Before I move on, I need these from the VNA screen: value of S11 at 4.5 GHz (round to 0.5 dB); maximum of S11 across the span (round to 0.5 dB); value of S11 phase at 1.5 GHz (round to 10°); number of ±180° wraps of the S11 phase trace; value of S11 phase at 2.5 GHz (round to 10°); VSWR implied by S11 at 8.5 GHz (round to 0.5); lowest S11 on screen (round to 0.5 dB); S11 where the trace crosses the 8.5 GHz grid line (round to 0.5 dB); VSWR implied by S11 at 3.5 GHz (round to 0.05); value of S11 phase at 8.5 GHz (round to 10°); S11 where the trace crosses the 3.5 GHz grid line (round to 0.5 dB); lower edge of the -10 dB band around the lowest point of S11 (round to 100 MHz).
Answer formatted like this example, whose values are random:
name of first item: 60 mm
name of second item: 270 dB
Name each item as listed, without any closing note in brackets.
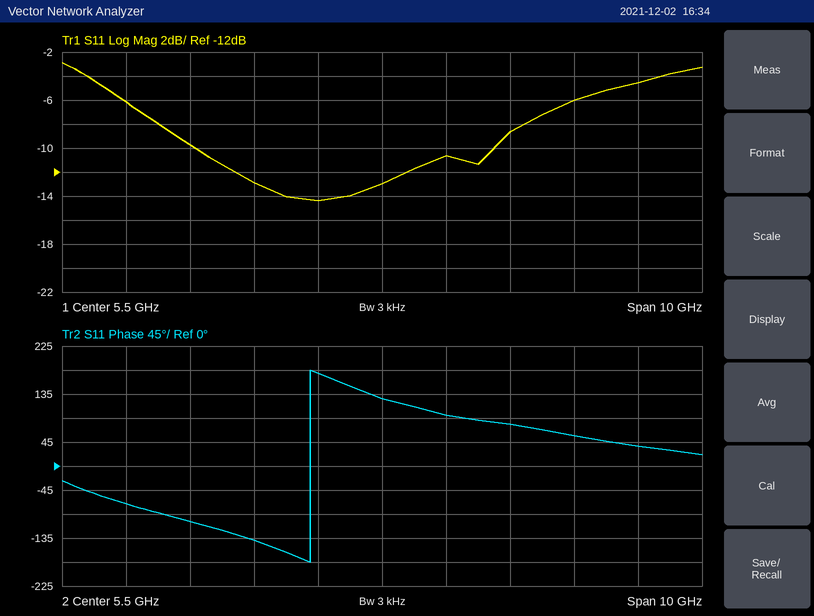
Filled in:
value of S11 at 4.5 GHz: -14.5 dB
maximum of S11 across the span: -3.0 dB
value of S11 phase at 1.5 GHz: -70°
number of ±180° wraps of the S11 phase trace: 1
value of S11 phase at 2.5 GHz: -100°
VSWR implied by S11 at 8.5 GHz: 3.0
lowest S11 on screen: -14.5 dB
S11 where the trace crosses the 8.5 GHz grid line: -6.0 dB
VSWR implied by S11 at 3.5 GHz: 1.60
value of S11 phase at 8.5 GHz: 60°
S11 where the trace crosses the 3.5 GHz grid line: -13.0 dB
lower edge of the -10 dB band around the lowest point of S11: 2.6 GHz
